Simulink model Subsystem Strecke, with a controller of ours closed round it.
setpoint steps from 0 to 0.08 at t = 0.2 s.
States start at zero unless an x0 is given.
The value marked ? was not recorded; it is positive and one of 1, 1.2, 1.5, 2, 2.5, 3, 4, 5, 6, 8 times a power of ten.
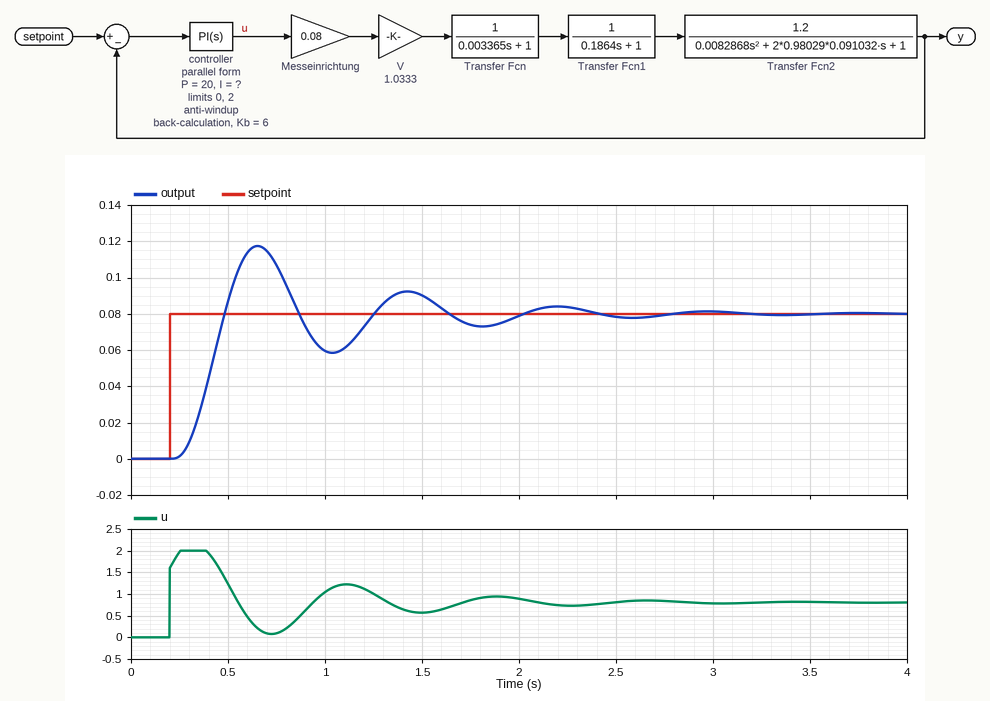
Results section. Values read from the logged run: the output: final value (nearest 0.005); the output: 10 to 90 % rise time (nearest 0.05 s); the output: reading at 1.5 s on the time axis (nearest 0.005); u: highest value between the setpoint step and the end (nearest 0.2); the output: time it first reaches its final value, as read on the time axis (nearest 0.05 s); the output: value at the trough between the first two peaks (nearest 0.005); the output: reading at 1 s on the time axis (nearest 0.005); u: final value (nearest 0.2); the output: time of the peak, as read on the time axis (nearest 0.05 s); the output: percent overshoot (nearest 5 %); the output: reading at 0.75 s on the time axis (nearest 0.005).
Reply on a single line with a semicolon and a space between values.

0.080; 0.15 s; 0.090; 2.0; 0.50 s; 0.060; 0.060; 0.8; 0.65 s; 45 %; 0.105
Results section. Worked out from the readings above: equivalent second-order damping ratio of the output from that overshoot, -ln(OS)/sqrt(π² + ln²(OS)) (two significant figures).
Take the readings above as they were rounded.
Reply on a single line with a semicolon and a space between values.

0.25
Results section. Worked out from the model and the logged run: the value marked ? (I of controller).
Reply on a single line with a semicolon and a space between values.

100
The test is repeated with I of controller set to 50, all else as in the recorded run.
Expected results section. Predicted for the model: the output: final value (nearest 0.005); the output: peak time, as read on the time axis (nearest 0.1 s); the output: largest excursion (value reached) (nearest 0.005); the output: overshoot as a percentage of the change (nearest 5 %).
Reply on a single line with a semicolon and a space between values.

0.080; 0.6 s; 0.095; 20 %
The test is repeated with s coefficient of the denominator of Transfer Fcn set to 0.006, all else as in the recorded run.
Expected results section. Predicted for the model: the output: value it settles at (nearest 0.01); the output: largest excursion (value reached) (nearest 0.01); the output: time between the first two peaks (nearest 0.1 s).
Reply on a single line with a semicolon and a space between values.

0.08; 0.12; 0.8 s
